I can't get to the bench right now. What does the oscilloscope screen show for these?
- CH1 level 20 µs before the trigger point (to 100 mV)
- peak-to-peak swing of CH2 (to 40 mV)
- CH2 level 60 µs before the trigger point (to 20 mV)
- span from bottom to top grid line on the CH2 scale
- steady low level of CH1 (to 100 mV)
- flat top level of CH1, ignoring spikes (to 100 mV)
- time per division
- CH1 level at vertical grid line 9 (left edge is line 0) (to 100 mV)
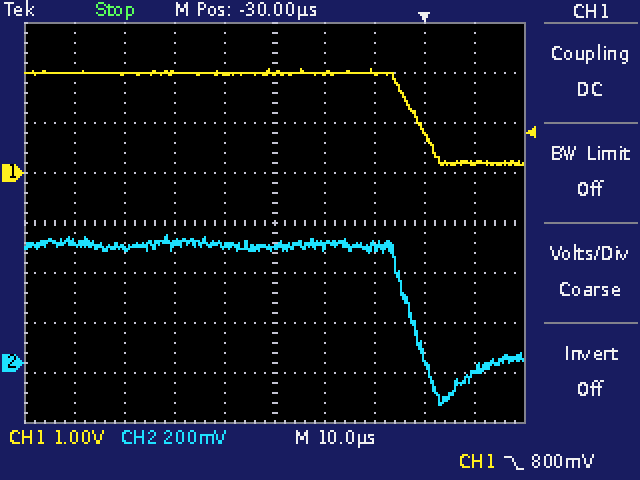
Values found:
2.0 V
680 mV
460 mV
1.6 V
200 mV
2.0 V
10 µs
200 mV
